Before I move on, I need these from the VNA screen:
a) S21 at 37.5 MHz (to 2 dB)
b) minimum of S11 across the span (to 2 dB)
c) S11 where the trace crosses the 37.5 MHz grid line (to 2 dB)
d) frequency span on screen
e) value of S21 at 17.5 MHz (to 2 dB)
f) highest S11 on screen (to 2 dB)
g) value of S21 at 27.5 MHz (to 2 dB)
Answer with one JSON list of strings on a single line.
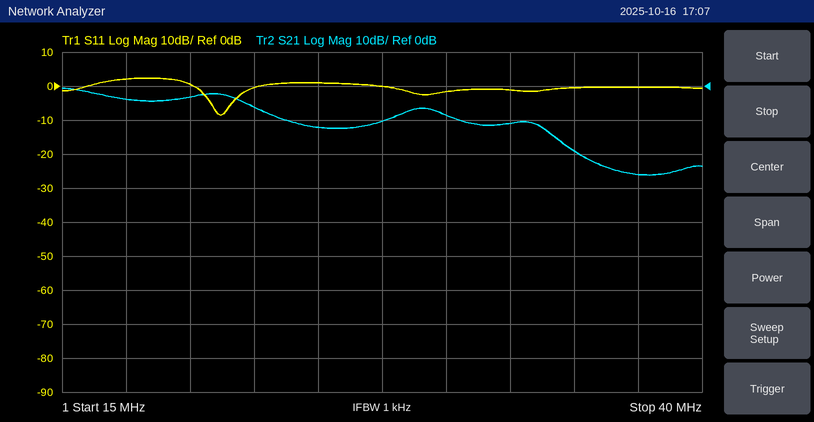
["-26 dB", "-8 dB", "0 dB", "25 MHz", "-4 dB", "2 dB", "-10 dB"]
